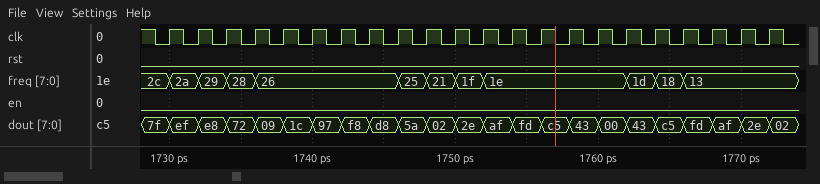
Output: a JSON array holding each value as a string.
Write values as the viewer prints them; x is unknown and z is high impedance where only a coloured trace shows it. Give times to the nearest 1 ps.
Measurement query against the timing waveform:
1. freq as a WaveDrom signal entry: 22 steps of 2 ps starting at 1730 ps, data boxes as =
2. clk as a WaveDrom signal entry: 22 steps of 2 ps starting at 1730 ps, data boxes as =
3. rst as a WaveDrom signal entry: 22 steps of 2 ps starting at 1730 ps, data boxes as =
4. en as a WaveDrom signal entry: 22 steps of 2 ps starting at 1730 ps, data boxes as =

["{name: 'freq', wave: '====....====....===...', data: '2a 29 28 26 25 21 1f 1e 1d 18 13'}", "{name: 'clk', wave: 'p.....................'}", "{name: 'rst', wave: '0.....................'}", "{name: 'en', wave: '0.....................'}"]
